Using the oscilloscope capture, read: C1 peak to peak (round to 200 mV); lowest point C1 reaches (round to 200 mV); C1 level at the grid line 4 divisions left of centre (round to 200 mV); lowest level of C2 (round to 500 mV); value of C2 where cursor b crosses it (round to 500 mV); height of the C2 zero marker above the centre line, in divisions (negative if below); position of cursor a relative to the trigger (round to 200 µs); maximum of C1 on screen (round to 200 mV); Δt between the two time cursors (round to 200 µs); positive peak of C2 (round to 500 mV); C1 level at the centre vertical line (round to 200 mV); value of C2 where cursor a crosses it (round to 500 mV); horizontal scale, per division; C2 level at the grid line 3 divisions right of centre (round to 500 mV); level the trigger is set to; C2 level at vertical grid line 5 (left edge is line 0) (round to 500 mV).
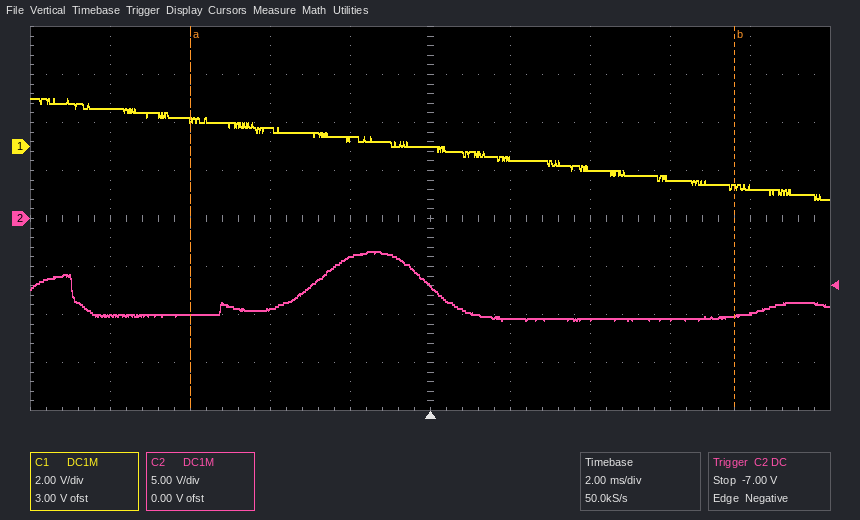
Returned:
4.2 V
-2.2 V
1.6 V
-10.5 V
-10.0 V
0.0 div
-6.0 ms
2.0 V
13.6 ms
-3.5 V
0.0 V
-10.0 V
2 ms
-10.5 V
-7.00 V
-7.0 V
